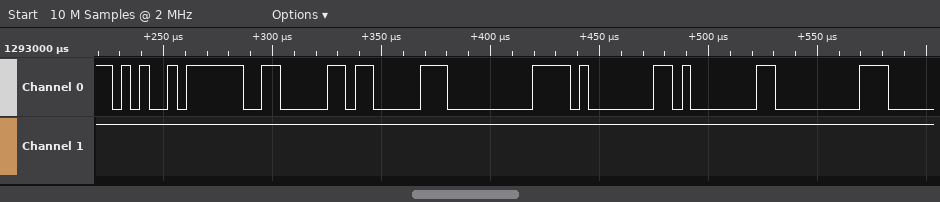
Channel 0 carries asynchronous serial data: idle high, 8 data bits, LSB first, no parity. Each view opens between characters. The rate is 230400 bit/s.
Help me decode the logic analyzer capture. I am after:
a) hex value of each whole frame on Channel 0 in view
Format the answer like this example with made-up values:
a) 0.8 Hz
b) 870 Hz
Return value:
a) A5, 06, 83, 00, 01, 01, 00
